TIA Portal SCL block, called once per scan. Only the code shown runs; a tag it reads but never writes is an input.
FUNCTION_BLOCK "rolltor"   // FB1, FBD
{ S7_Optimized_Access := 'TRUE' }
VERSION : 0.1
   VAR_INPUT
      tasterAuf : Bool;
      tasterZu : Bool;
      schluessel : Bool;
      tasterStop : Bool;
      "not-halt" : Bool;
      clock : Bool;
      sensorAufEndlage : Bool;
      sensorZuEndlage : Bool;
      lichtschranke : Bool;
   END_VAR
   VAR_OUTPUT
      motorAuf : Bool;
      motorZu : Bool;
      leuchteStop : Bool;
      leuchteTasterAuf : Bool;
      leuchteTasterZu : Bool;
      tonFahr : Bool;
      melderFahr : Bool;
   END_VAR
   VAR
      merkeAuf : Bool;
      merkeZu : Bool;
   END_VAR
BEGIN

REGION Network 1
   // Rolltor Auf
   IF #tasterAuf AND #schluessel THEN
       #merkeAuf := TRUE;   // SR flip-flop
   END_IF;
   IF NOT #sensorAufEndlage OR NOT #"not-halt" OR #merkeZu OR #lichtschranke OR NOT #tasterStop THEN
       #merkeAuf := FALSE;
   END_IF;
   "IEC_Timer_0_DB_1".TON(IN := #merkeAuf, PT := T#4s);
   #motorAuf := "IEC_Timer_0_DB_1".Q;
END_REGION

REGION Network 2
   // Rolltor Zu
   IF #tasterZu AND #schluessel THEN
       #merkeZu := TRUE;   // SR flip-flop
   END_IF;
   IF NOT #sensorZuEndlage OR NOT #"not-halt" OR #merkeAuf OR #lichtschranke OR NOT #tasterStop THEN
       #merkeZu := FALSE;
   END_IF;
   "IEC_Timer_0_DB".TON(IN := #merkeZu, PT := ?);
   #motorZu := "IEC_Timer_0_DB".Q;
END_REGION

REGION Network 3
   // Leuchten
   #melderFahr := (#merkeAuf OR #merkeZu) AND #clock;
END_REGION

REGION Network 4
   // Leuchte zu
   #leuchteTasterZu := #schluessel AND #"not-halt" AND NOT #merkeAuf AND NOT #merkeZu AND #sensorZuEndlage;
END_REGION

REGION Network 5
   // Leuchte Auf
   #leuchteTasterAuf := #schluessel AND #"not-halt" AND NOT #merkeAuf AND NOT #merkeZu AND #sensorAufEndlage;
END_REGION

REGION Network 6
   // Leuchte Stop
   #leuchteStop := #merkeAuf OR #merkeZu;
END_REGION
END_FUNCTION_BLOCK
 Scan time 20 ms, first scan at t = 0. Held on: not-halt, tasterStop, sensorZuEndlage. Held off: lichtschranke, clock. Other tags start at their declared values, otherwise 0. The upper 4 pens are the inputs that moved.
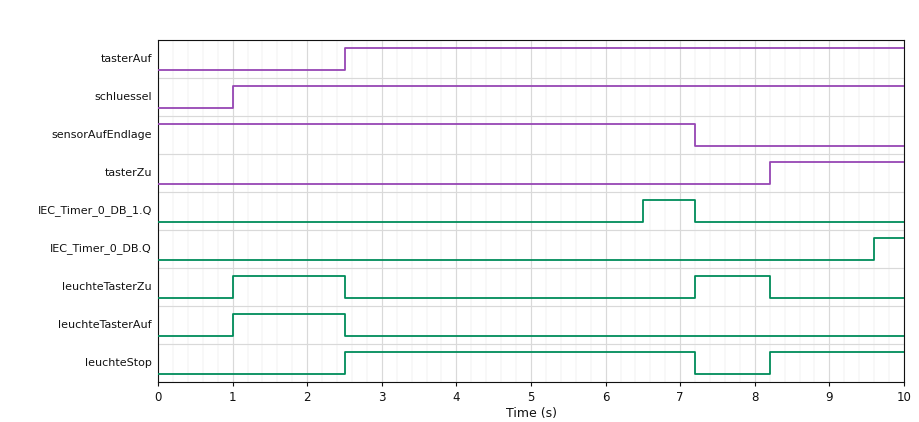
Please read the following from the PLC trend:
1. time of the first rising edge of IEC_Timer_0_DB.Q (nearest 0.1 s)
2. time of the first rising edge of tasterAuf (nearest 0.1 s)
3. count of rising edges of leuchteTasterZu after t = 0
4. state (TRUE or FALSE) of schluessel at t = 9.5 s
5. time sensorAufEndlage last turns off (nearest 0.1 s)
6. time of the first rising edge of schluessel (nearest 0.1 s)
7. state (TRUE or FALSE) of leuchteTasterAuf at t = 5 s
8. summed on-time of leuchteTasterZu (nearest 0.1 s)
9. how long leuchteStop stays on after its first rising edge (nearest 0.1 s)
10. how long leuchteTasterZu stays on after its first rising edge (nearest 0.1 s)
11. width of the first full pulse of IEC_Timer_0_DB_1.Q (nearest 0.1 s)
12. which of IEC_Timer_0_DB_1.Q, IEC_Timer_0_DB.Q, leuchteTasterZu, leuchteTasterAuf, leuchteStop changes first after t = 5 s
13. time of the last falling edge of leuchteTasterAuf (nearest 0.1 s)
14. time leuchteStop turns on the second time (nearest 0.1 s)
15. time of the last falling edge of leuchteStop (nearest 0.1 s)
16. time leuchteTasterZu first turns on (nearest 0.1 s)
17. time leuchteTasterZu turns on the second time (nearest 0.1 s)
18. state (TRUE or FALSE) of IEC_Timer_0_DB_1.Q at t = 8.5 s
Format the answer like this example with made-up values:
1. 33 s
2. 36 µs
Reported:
1. 9.6 s
2. 2.5 s
3. 2
4. TRUE
5. 7.2 s
6. 1.0 s
7. FALSE
8. 2.5 s
9. 4.7 s
10. 1.5 s
11. 0.7 s
12. IEC_Timer_0_DB_1.Q
13. 2.5 s
14. 8.2 s
15. 7.2 s
16. 1.0 s
17. 7.2 s
18. FALSE
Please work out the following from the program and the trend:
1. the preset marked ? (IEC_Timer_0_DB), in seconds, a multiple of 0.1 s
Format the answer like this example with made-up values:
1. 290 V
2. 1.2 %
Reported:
1. 1.4 s
